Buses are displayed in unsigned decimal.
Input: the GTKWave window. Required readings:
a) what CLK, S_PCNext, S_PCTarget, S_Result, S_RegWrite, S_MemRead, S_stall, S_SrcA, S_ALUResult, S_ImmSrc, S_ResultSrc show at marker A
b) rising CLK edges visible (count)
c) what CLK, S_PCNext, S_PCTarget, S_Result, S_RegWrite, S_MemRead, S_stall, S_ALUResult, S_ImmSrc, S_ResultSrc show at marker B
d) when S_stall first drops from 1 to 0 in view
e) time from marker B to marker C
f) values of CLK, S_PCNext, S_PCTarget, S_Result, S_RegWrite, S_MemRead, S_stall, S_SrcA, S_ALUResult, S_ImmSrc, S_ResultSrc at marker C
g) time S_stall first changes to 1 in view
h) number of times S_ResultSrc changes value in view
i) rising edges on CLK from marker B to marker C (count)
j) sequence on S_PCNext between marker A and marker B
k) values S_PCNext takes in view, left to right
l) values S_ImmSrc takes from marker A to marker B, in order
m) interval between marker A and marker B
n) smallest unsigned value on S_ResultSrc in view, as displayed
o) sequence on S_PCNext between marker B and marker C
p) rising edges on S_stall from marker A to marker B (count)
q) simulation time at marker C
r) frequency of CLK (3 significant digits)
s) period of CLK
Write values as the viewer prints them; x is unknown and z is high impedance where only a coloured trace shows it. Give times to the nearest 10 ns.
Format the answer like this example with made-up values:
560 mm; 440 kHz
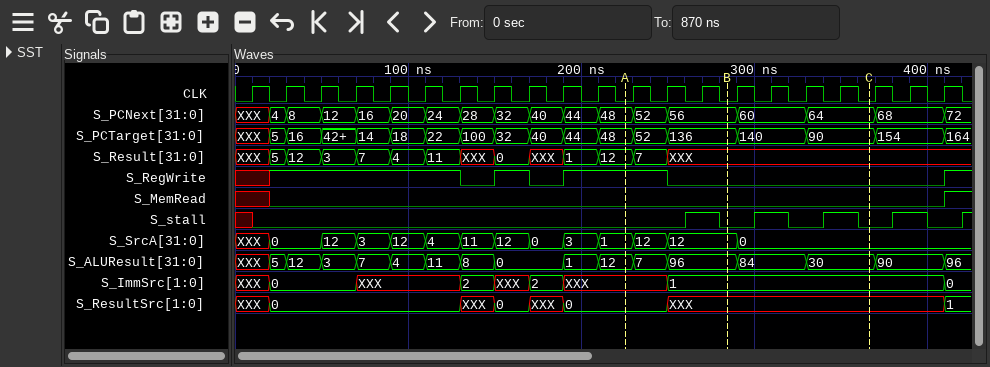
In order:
CLK=0, S_PCNext=48, S_PCTarget=48, S_Result=12, S_RegWrite=1, S_MemRead=0, S_stall=0, S_SrcA=1, S_ALUResult=12, S_ImmSrc=XXX, S_ResultSrc=0; 21; CLK=0, S_PCNext=56, S_PCTarget=136, S_Result=XXX, S_RegWrite=0, S_MemRead=0, S_stall=0, S_ALUResult=96, S_ImmSrc=1, S_ResultSrc=XXX; 280 ns; 80 ns; CLK=0, S_PCNext=64, S_PCTarget=90, S_Result=XXX, S_RegWrite=0, S_MemRead=0, S_stall=0, S_SrcA=0, S_ALUResult=30, S_ImmSrc=1, S_ResultSrc=XXX; 260 ns; 7; 4; 48, 52, 56; XXX, 4, 8, 12, 16, 20, 24, 28, 32, 40, 44, 48, 52, 56, 60, 64, 68, 72; XXX, 1; 60 ns; 0; 56, 60, 64; 1; 370 ns; 50.0 MHz; 20 ns
